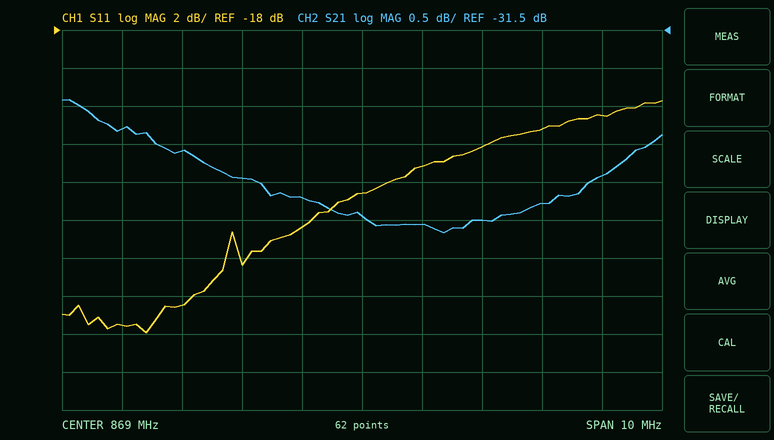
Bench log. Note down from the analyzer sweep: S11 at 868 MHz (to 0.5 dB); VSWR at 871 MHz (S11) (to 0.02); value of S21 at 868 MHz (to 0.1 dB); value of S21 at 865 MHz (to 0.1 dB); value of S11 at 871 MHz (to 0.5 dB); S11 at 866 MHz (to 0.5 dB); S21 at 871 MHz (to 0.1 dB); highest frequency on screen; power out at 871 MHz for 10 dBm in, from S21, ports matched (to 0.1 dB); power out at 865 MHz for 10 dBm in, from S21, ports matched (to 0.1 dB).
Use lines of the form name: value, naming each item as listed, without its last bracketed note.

S11 at 868 MHz: -28.5 dB
VSWR at 871 MHz (S11): 1.14
value of S21 at 868 MHz: -33.7 dB
value of S21 at 865 MHz: -32.8 dB
value of S11 at 871 MHz: -24.0 dB
S11 at 866 MHz: -32.5 dB
S21 at 871 MHz: -34.0 dB
highest frequency on screen: 874 MHz
power out at 871 MHz for 10 dBm in, from S21, ports matched: -24.0 dBm
power out at 865 MHz for 10 dBm in, from S21, ports matched: -22.8 dBm
